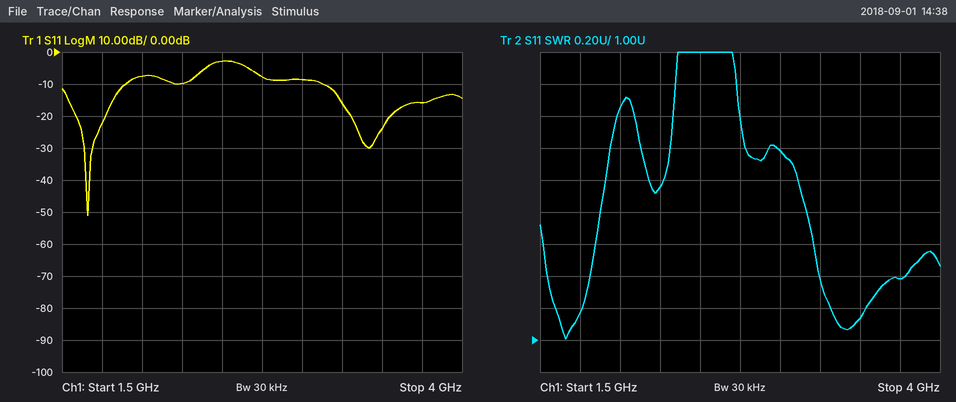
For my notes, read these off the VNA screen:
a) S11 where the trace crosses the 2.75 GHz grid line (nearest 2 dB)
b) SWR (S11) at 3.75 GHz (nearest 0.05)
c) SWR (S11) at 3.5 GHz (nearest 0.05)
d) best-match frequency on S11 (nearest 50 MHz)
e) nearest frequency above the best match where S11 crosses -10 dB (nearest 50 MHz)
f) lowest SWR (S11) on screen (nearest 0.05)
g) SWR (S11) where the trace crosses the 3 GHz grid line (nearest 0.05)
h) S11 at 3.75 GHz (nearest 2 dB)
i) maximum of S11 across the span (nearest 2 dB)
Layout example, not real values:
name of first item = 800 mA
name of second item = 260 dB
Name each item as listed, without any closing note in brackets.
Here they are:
S11 where the trace crosses the 2.75 GHz grid line = -8 dB
SWR (S11) at 3.75 GHz = 1.40
SWR (S11) at 3.5 GHz = 1.15
best-match frequency on S11 = 1.65 GHz
nearest frequency above the best match where S11 crosses -10 dB = 1.90 GHz
lowest SWR (S11) on screen = 1.00
SWR (S11) where the trace crosses the 3 GHz grid line = 2.20
S11 at 3.75 GHz = -16 dB
maximum of S11 across the span = -2 dB
